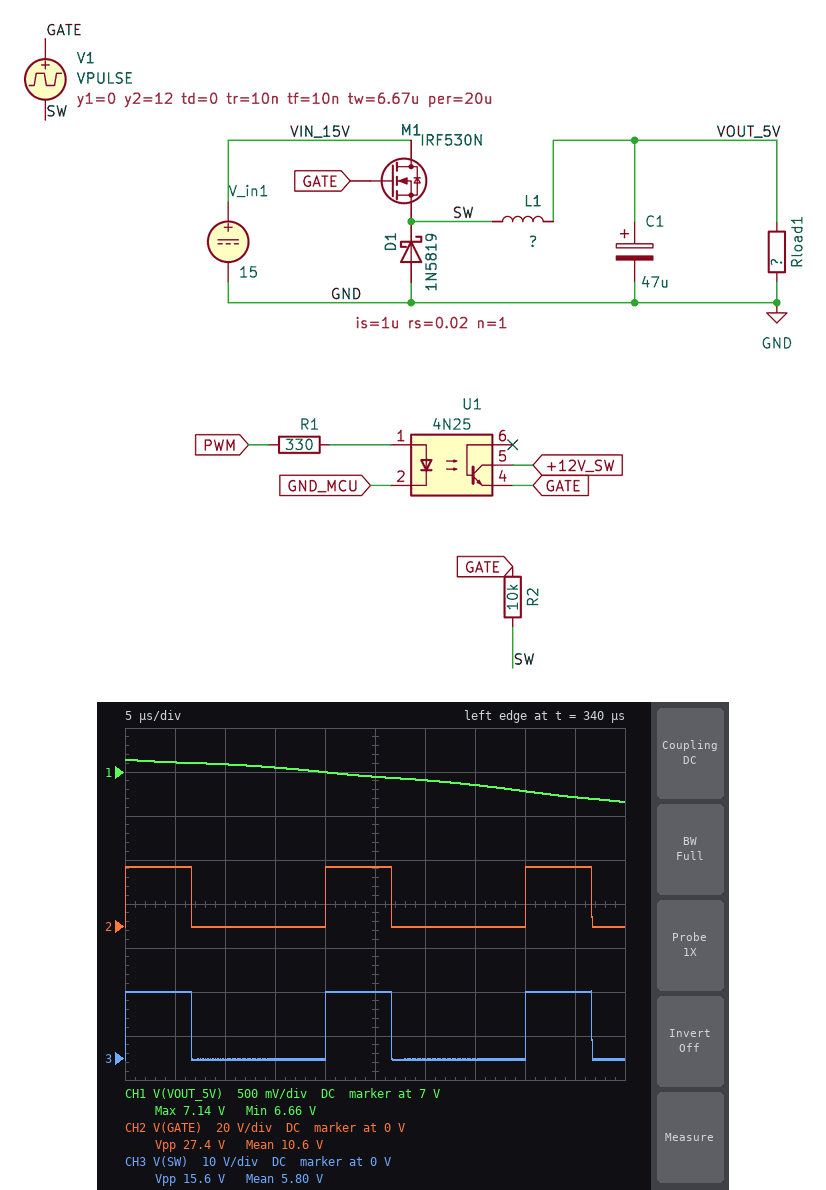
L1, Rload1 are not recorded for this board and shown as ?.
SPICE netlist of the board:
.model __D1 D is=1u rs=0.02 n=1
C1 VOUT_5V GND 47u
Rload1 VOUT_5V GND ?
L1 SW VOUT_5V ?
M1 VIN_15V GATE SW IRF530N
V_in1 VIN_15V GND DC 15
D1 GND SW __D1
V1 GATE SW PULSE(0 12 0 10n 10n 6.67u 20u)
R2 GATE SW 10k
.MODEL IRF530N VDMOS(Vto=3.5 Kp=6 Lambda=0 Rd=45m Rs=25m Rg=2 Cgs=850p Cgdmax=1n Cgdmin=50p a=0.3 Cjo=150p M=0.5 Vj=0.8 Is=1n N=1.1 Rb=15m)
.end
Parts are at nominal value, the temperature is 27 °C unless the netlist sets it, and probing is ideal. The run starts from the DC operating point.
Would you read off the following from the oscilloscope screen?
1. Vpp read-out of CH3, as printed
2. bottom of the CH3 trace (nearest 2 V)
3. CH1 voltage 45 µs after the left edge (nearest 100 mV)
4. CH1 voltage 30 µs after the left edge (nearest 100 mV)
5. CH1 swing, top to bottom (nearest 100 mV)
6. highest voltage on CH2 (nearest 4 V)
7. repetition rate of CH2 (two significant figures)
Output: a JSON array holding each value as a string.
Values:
["15.6 V", "0 V", "6.7 V", "6.9 V", "500 mV", "28 V", "50 kHz"]
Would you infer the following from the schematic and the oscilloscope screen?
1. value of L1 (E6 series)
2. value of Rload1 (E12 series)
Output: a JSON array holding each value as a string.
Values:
["220 µH", "5.6 Ω"]
